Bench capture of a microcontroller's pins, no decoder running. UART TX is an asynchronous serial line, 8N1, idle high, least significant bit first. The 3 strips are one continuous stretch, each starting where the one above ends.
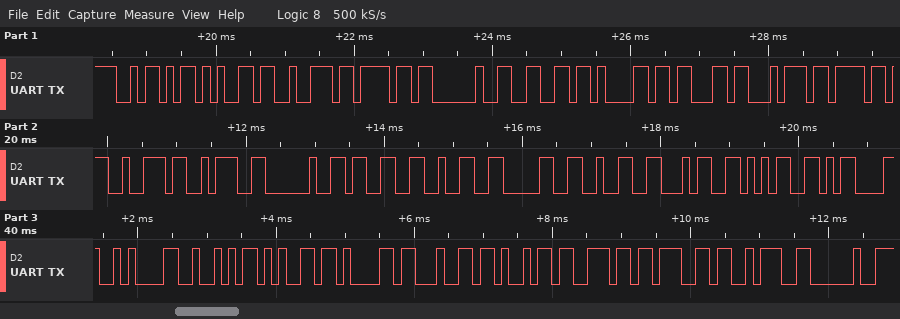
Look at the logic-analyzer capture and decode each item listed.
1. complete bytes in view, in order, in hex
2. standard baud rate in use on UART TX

0x5A 0x65 0x72 0x6F 0x20 0x66 0x61 0x63 0x74 0x6F 0x72 0x3A 0x20 0x33 0x32 0x30 0x32 0x34 0x35 0x0D 0x0A 0x52 0x65 0x61 0x64 0x69 0x6E 0x67 0x3A 0x20
9600 baud
